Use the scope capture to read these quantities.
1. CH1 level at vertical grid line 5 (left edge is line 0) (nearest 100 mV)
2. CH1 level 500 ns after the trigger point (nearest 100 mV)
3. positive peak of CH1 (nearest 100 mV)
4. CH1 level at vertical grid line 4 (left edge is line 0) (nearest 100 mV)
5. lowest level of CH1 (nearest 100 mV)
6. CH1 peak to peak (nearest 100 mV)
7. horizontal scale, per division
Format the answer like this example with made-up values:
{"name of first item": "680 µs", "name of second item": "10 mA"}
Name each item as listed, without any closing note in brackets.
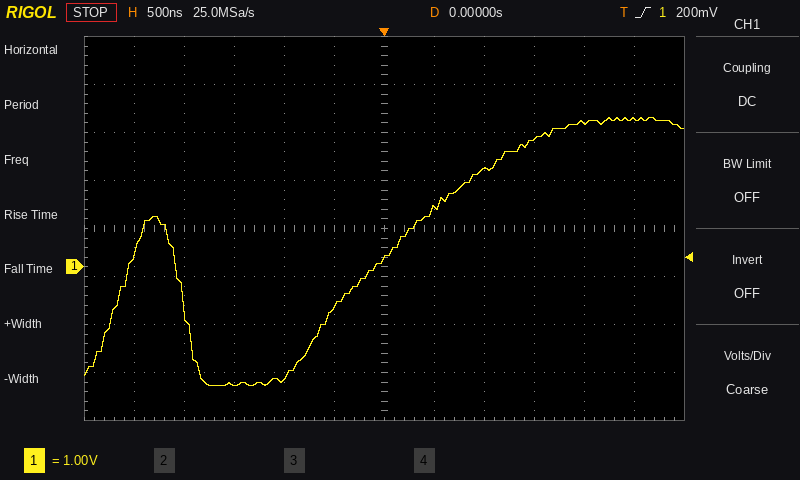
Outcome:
{"CH1 level at vertical grid line 5 (left edge is line 0)": "-800 mV", "CH1 level 500 ns after the trigger point": "1.2 V", "positive peak of CH1": "3.1 V", "CH1 level at vertical grid line 4 (left edge is line 0)": "-2.3 V", "lowest level of CH1": "-2.5 V", "CH1 peak to peak": "5.6 V", "horizontal scale, per division": "500 ns"}
